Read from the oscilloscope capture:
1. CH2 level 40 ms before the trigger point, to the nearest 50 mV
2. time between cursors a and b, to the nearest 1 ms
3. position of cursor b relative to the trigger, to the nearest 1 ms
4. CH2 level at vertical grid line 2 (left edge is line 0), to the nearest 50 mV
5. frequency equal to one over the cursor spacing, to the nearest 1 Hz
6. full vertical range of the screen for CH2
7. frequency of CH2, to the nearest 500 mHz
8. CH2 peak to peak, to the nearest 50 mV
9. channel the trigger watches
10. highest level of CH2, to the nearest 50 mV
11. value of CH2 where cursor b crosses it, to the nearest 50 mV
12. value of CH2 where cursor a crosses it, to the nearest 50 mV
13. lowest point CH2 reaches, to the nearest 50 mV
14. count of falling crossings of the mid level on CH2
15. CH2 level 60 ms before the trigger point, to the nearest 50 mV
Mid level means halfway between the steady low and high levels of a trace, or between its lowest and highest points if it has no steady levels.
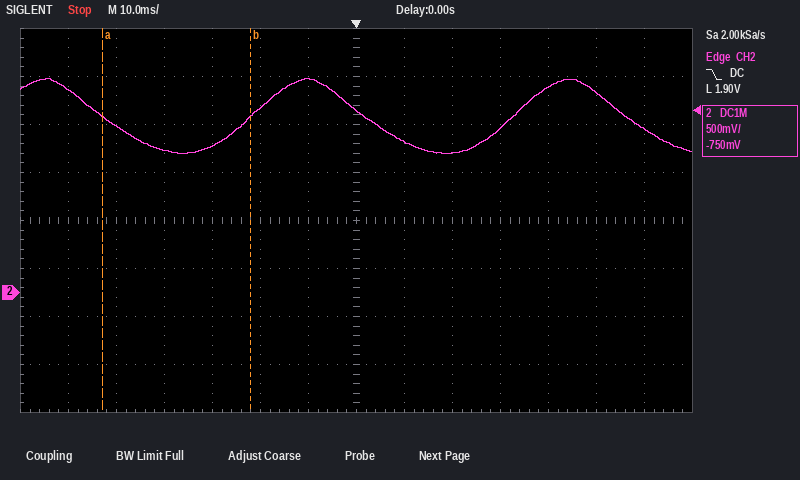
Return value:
1.50 V
31 ms
-22 ms
1.75 V
32 Hz
4 V
18.5 Hz
800 mV
CH2
2.25 V
1.85 V
1.85 V
1.45 V
3
2.10 V
